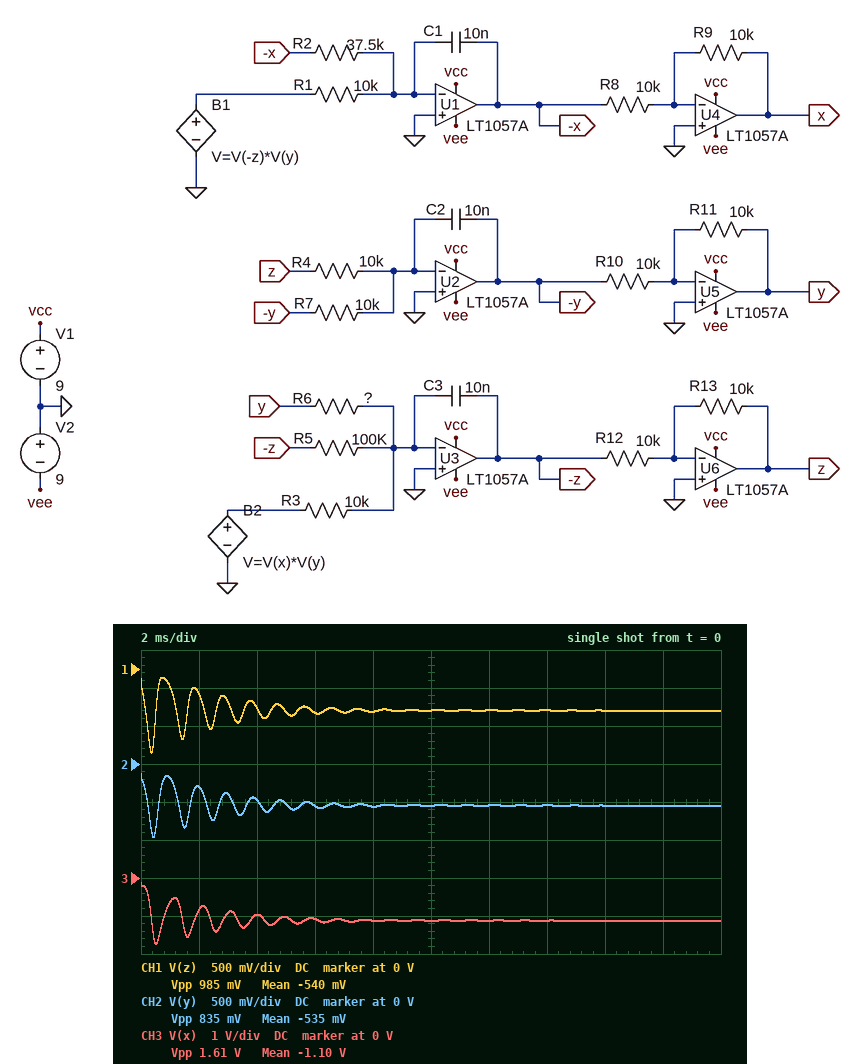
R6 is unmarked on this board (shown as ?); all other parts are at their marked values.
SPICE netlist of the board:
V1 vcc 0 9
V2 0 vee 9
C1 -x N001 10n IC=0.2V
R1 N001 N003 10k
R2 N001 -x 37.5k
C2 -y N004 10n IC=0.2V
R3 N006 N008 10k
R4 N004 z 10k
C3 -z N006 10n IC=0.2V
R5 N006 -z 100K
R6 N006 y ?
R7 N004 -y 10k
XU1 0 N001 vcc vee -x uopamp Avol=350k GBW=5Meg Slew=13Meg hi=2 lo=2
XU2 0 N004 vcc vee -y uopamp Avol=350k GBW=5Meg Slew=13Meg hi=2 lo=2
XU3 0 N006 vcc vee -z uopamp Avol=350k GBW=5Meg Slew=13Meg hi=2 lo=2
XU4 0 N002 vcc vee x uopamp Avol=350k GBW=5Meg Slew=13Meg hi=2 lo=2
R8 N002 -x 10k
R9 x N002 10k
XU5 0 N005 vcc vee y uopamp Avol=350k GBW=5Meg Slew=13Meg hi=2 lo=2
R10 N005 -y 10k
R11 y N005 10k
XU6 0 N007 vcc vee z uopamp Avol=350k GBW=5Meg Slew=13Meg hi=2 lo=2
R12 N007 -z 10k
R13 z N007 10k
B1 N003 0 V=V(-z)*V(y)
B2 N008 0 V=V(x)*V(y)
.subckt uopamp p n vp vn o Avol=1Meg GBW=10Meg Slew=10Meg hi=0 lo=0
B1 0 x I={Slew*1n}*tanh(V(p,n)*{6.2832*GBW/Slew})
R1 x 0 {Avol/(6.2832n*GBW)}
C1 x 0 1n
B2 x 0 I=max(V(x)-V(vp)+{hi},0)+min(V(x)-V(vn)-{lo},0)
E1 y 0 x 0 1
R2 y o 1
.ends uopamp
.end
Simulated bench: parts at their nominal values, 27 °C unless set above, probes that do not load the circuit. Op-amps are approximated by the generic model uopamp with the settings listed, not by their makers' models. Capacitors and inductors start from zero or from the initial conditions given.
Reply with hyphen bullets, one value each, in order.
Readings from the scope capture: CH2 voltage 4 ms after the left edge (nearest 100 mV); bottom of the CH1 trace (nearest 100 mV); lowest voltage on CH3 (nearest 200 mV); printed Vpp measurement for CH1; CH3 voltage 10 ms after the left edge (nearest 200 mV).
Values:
- -500 mV
- -1.1 V
- -1.8 V
- 985 mV
- -1.2 V
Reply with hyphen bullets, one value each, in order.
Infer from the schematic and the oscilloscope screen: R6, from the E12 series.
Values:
- 8.2 kΩ
